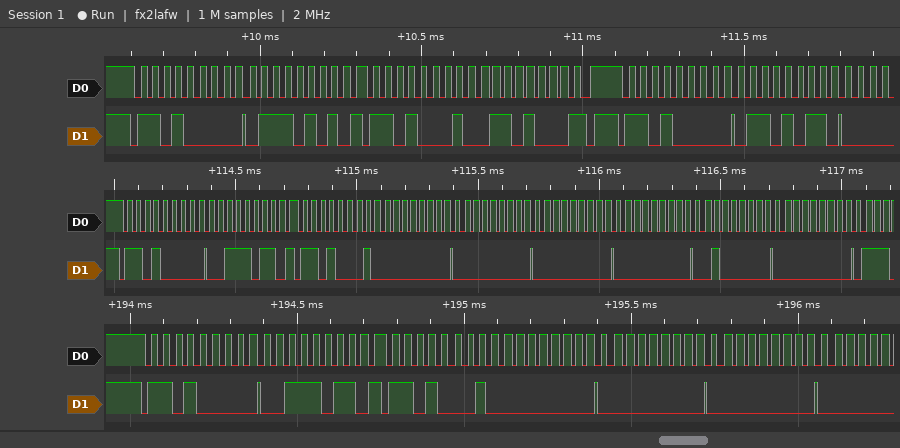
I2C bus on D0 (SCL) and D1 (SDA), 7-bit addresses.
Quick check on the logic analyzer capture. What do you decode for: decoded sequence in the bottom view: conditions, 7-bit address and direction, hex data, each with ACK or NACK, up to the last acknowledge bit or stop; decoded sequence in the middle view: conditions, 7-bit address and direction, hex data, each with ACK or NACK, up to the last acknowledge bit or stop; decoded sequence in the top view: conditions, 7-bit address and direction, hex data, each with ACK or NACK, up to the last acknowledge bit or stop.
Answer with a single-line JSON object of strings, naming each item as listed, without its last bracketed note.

{"decoded sequence in the bottom view: conditions, 7-bit address and direction, hex data, each with ACK or NACK, up to the last acknowledge bit or stop": "start, address 68 write ACK, 3B ACK, repeated start, address 68 read ACK, 00 ACK, 00 ACK, 00 ACK", "decoded sequence in the middle view: conditions, 7-bit address and direction, hex data, each with ACK or NACK, up to the last acknowledge bit or stop": "start, address 68 write ACK, 3B ACK, repeated start, address 68 read ACK, 00 ACK, 00 ACK, 00 ACK, 00 ACK, 40 ACK, 00 ACK", "decoded sequence in the top view: conditions, 7-bit address and direction, hex data, each with ACK or NACK, up to the last acknowledge bit or stop": "start, address 68 write ACK, 75 ACK, repeated start, address 68 read ACK, 68 NACK, stop, start, address 68 write ACK, 6B ACK"}
